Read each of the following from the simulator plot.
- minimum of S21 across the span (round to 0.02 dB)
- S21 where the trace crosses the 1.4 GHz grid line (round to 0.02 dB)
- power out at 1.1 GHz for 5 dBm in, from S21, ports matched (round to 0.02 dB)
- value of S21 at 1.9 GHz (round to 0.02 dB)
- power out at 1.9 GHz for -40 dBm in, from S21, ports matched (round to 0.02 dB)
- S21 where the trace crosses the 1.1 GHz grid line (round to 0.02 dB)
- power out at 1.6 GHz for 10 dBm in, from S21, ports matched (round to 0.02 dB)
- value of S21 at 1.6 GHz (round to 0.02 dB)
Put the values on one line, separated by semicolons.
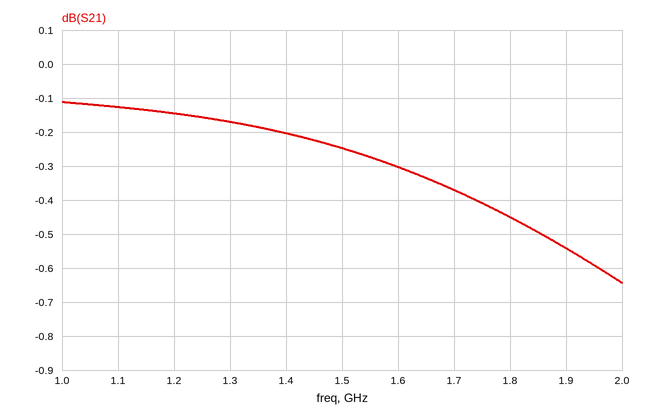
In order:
-0.64 dB; -0.20 dB; 4.88 dBm; -0.54 dB; -40.54 dBm; -0.12 dB; 9.70 dBm; -0.30 dB
